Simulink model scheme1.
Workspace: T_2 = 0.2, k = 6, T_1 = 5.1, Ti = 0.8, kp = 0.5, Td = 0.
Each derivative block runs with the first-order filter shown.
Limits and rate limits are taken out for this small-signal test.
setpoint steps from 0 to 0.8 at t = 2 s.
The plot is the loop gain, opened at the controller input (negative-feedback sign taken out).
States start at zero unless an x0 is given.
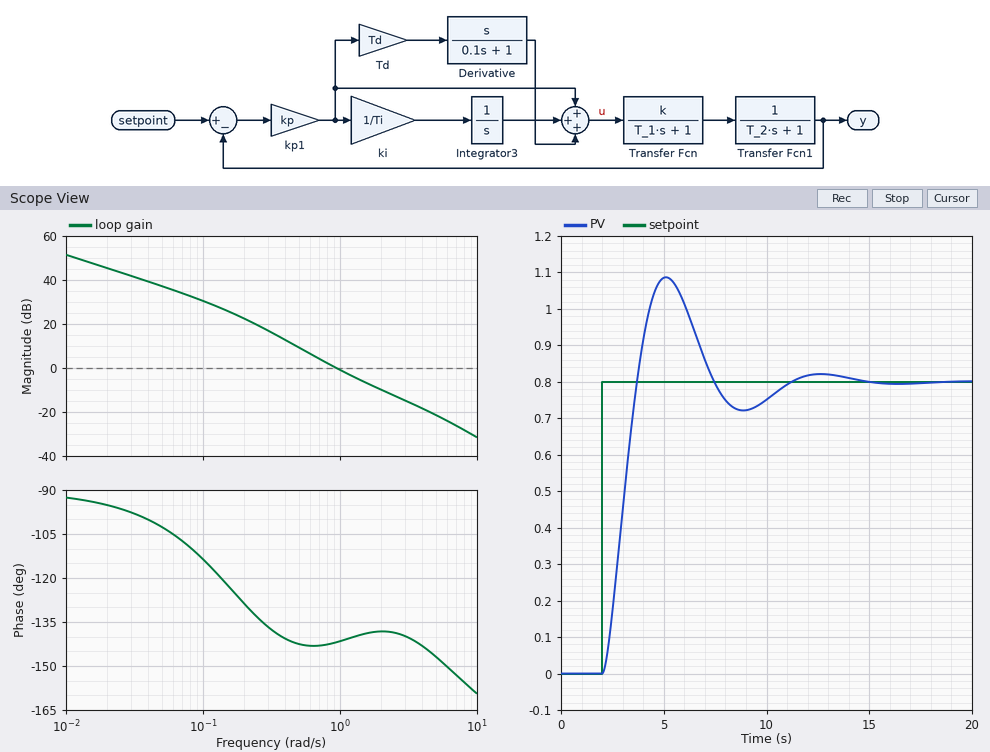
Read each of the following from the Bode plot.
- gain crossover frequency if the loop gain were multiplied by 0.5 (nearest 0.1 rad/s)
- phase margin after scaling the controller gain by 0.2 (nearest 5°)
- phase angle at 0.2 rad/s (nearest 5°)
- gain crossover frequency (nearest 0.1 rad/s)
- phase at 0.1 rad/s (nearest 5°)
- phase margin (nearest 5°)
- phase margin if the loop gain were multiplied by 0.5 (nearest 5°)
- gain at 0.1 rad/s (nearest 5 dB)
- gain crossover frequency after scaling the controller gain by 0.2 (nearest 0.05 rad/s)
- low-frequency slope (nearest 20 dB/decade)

0.6 rad/s
40°
-130°
0.9 rad/s
-115°
40°
35°
30 dB
0.35 rad/s
-20 dB/decade
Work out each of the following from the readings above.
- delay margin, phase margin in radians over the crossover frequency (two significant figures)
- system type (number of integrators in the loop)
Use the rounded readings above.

0.78 s
1
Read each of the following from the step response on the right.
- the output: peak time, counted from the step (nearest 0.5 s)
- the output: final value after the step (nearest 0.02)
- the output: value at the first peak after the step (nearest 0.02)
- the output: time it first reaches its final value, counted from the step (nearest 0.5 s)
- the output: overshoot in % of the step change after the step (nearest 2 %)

3.0 s
0.80
1.08
1.5 s
36 %
